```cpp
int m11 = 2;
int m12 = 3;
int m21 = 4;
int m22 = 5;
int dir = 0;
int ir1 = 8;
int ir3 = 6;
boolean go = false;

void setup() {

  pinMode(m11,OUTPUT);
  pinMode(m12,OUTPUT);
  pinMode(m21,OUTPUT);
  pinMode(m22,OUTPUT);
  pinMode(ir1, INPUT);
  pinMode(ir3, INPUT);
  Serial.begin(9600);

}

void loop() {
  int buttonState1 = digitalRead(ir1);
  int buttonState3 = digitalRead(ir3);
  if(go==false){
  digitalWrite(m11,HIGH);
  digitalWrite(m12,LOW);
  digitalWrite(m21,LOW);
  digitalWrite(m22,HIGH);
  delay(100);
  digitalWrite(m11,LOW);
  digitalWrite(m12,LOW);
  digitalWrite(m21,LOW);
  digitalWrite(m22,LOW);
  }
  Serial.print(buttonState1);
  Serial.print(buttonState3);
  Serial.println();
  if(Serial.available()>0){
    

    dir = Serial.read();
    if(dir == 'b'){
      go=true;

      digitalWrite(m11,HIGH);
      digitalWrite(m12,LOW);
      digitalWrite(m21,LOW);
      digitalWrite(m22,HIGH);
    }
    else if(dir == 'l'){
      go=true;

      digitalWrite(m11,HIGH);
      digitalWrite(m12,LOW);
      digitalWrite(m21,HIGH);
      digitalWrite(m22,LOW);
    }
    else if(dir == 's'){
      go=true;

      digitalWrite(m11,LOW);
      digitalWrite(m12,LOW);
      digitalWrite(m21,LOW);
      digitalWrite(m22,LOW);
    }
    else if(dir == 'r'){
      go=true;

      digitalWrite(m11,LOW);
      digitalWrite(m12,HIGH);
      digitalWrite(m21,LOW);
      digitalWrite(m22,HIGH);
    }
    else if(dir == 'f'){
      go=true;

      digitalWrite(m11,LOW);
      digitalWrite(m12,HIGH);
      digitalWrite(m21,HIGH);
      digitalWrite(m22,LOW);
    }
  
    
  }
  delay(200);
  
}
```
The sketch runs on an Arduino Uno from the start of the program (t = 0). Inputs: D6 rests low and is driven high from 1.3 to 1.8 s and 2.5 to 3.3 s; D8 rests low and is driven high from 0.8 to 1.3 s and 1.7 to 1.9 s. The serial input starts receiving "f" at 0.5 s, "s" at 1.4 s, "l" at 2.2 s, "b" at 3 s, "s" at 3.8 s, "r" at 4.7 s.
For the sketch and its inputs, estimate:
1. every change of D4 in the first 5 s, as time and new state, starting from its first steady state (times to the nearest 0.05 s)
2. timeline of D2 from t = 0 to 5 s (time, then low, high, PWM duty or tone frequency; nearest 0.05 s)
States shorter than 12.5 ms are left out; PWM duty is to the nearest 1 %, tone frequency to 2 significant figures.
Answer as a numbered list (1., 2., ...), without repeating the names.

1. 0 s low; 0.7 s high; 1.5 s low; 2.3 s high; 3.1 s low
2. 0 s high; 0.1 s low; 0.3 s high; 0.4 s low; 0.6 s high; 0.7 s low; 2.3 s high; 3.9 s low
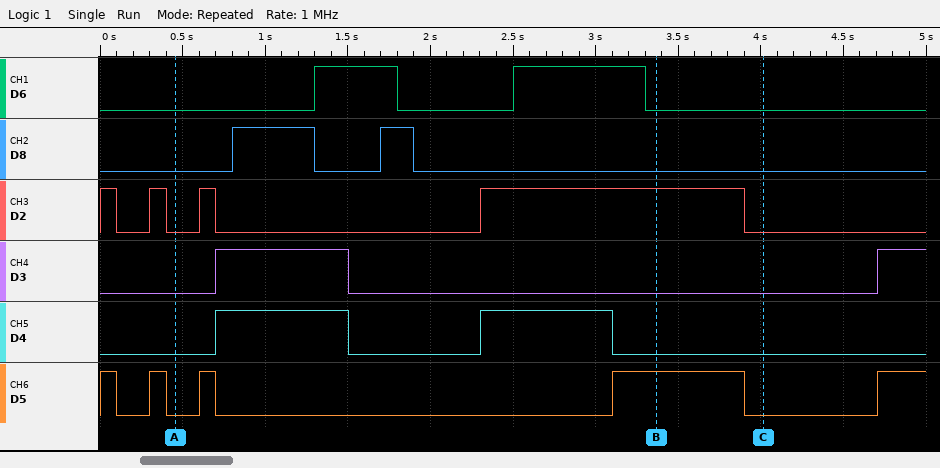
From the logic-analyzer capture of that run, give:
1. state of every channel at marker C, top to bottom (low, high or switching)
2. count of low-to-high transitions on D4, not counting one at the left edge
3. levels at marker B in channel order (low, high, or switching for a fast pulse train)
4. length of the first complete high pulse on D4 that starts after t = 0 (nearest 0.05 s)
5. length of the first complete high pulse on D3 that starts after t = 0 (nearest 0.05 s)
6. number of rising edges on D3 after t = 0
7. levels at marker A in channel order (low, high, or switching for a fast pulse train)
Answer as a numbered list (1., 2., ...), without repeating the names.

1. D6 low, D8 low, D2 low, D3 low, D4 low, D5 low
2. 2
3. D6 low, D8 low, D2 high, D3 low, D4 low, D5 high
4. 0.80 s
5. 0.80 s
6. 2
7. D6 low, D8 low, D2 low, D3 low, D4 low, D5 low
